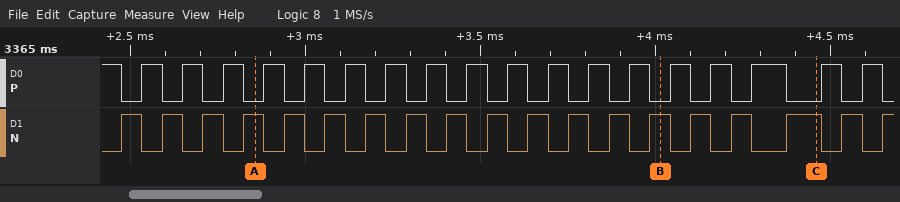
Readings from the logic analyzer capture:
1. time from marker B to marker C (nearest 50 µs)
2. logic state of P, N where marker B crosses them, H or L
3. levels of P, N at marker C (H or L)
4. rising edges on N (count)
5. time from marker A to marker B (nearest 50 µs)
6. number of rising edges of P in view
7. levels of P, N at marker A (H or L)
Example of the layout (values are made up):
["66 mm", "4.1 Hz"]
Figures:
["450 µs", "P=L, N=H", "P=L, N=H", "19", "1150 µs", "18", "P=L, N=H"]
